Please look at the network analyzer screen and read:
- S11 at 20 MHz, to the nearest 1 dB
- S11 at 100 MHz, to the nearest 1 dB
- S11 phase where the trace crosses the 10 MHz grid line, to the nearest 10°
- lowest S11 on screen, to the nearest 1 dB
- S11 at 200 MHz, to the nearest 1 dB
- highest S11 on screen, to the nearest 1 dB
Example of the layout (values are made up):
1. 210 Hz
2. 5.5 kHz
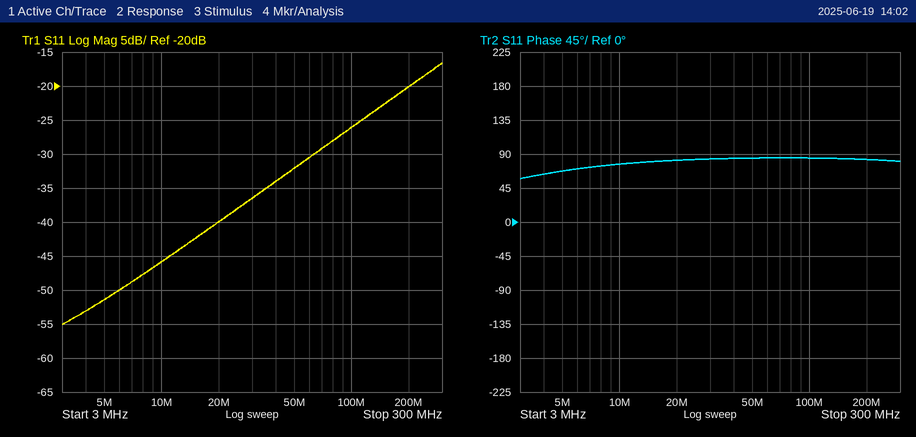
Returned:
1. -40 dB
2. -26 dB
3. 80°
4. -55 dB
5. -20 dB
6. -17 dB
